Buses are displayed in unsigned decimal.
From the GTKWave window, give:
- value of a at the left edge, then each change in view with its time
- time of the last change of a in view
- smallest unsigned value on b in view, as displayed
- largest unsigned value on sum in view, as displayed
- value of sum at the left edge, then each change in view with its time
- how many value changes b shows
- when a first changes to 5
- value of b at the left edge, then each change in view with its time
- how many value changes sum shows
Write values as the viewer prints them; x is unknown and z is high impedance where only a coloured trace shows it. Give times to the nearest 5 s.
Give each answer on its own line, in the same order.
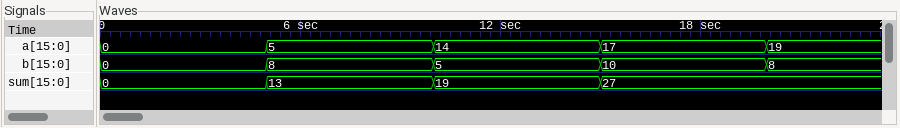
0, 5 at 5 s, 14 at 10 s, 17 at 15 s, 19 at 20 s
20 s
0
27
0, 13 at 5 s, 19 at 10 s, 27 at 15 s
4
5 s
0, 8 at 5 s, 5 at 10 s, 10 at 15 s, 8 at 20 s
3
